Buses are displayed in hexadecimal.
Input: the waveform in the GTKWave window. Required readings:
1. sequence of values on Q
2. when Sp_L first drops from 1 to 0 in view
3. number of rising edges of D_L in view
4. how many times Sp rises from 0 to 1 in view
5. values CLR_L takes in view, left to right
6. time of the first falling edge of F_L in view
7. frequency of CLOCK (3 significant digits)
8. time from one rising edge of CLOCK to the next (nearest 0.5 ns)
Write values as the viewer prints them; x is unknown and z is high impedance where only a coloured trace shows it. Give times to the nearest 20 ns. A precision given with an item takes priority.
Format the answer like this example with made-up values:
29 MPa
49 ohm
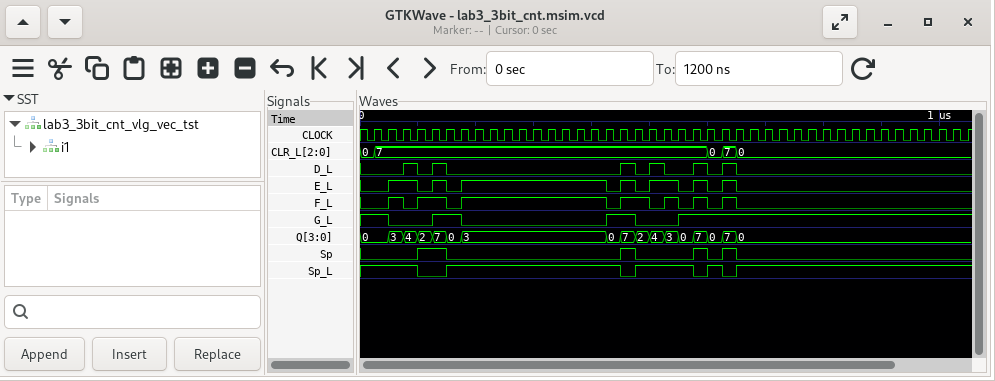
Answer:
0, 3, 4, 2, 7, 0, 3, 0, 7, 2, 4, 3, 0, 7, 0, 7, 0
100 ns
6
4
0, 7, 0, 7, 0
80 ns
40.0 MHz
25 ns
